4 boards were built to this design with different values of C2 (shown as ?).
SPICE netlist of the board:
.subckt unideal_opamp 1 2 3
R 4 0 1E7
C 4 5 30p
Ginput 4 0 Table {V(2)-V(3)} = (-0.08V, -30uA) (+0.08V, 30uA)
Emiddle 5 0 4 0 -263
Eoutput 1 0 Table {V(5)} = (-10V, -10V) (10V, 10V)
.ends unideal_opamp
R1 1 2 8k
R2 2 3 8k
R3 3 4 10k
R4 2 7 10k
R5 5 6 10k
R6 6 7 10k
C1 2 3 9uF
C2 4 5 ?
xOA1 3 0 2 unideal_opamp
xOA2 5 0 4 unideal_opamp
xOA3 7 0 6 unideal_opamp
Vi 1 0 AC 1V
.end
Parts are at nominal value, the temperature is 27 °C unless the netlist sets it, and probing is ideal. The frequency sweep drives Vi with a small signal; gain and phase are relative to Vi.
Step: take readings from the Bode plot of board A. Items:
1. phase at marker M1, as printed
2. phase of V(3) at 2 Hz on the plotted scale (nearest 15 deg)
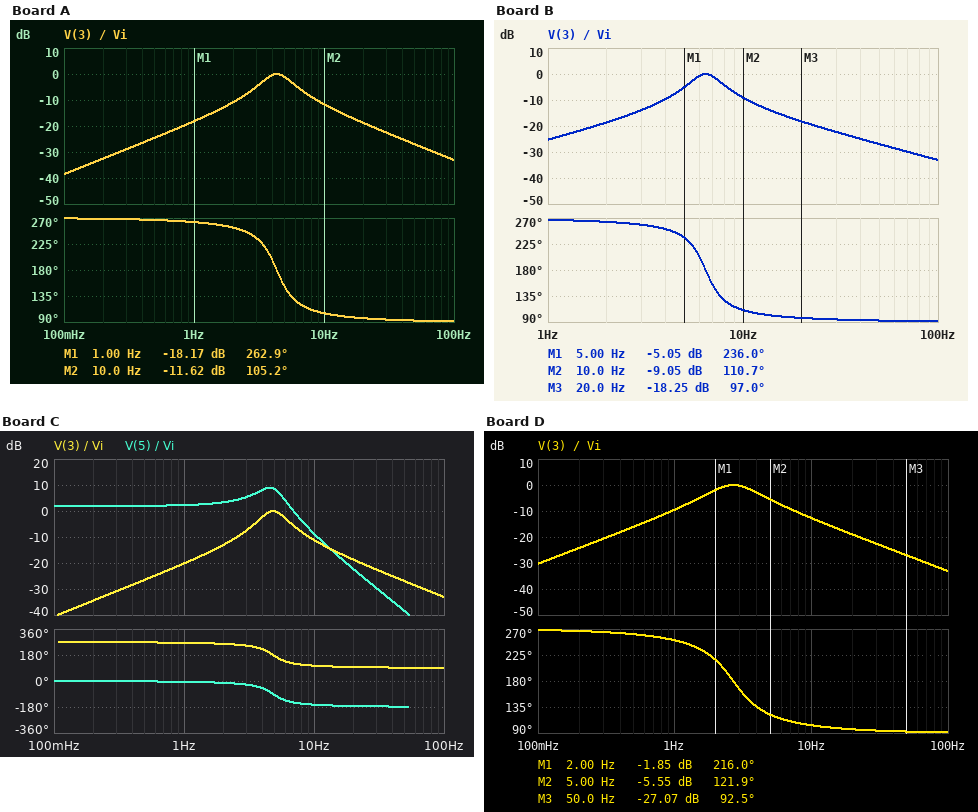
262.9 deg
255 deg
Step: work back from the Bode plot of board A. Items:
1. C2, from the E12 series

1.5 µF
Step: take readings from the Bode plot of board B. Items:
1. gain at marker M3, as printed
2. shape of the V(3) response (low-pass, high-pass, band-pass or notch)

-18.25 dB
band-pass
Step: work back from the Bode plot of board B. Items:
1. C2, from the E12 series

680 nF
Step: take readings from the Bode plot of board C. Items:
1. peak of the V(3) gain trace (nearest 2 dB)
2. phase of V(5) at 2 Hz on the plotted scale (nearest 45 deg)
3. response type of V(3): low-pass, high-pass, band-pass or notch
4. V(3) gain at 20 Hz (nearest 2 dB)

0 dB
0 deg
band-pass
-18 dB
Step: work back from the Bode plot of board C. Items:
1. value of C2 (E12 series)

1.2 µF
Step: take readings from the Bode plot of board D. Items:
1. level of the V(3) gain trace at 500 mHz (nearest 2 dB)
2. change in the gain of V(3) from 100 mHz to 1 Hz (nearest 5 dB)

-16 dB
20 dB
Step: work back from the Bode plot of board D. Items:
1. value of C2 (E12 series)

3.9 µF
